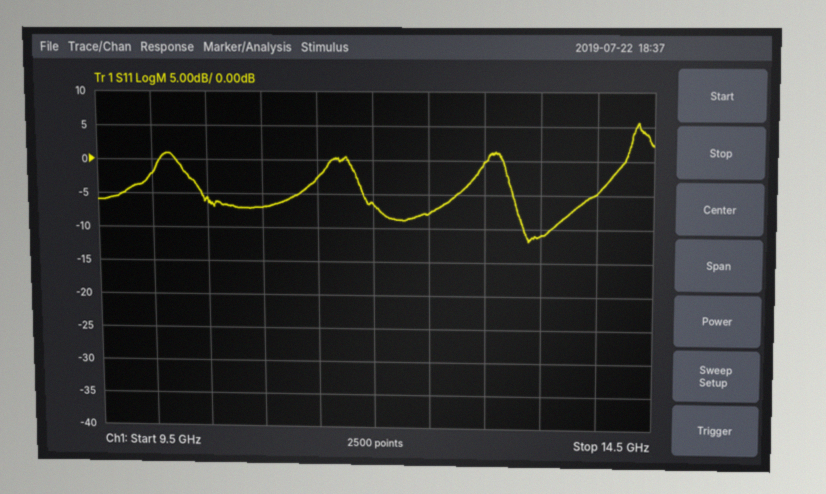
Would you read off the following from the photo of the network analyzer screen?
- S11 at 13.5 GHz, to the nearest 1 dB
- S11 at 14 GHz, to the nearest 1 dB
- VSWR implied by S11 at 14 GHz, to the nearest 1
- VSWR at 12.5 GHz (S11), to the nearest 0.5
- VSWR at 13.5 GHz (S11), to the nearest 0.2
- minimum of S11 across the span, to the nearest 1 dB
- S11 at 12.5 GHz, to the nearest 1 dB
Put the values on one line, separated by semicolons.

-11 dB; -5 dB; 4; 2.5; 1.8; -12 dB; -8 dB
